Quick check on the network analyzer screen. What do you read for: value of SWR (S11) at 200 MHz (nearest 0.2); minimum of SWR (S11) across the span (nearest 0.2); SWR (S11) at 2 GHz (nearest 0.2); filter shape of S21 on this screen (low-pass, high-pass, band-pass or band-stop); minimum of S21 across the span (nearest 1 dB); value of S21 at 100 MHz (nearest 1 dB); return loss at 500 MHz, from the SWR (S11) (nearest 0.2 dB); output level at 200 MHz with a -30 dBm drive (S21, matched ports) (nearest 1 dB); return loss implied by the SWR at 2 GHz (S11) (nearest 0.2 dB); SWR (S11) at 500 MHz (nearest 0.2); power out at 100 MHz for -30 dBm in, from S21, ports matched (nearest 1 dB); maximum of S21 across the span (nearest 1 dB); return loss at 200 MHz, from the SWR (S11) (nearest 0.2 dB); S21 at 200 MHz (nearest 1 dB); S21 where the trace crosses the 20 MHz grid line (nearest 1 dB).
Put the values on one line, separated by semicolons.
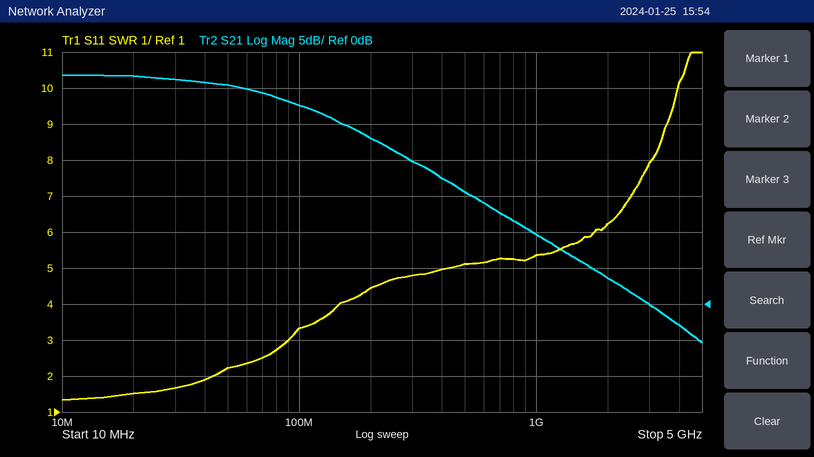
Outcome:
4.4; 1.4; 6.2; low-pass; -5 dB; 28 dB; 3.4 dB; -7 dBm; 2.8 dB; 5.2; -2 dBm; 32 dB; 4.0 dB; 23 dB; 32 dB
